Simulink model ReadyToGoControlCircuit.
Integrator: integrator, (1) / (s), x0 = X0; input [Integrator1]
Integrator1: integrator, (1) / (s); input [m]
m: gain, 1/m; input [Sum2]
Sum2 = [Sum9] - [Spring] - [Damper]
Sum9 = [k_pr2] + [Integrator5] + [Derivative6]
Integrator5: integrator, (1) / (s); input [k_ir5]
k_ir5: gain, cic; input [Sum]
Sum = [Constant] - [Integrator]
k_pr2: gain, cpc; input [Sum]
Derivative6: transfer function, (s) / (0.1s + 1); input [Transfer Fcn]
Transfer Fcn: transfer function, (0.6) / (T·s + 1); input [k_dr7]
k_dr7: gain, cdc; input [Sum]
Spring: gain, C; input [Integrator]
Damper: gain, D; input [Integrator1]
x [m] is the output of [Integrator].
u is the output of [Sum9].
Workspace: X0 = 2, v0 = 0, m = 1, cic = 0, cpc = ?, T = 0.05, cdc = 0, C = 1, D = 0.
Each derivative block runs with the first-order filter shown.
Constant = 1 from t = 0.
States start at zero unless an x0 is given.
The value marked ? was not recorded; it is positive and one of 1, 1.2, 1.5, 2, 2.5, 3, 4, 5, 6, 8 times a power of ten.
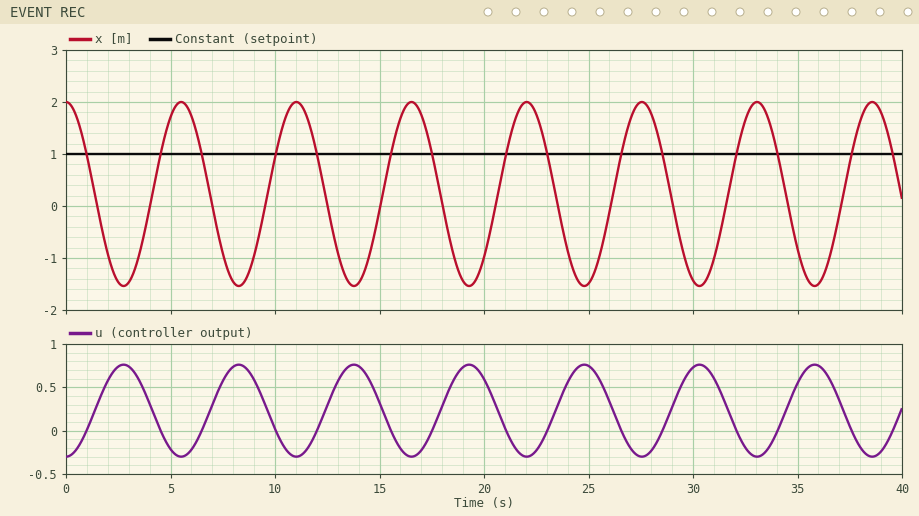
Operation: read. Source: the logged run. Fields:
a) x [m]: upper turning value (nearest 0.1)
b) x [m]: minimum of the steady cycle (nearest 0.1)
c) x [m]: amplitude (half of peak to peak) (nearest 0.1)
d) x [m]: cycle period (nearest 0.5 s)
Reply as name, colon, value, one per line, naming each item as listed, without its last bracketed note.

x [m]: upper turning value: 2.0
x [m]: minimum of the steady cycle: -1.5
x [m]: amplitude (half of peak to peak): 1.8
x [m]: cycle period: 5.5 s
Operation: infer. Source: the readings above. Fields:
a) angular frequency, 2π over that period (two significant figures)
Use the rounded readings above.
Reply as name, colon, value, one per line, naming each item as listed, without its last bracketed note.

angular frequency, 2π over that period: 1.1 rad/s
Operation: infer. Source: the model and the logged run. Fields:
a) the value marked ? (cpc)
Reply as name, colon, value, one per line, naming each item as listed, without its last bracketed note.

the value marked ?: 0.3
